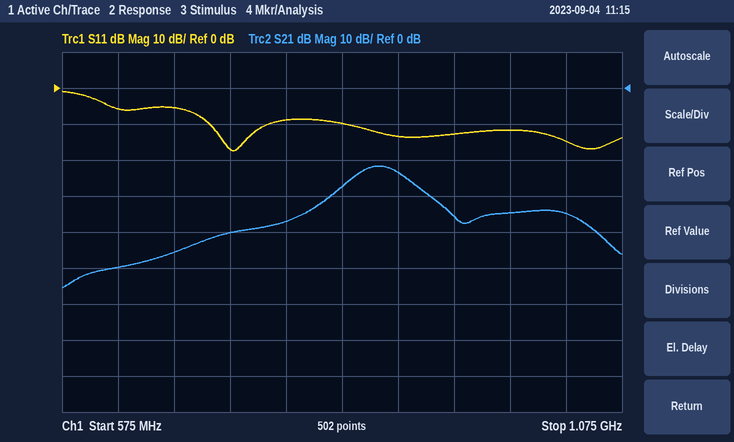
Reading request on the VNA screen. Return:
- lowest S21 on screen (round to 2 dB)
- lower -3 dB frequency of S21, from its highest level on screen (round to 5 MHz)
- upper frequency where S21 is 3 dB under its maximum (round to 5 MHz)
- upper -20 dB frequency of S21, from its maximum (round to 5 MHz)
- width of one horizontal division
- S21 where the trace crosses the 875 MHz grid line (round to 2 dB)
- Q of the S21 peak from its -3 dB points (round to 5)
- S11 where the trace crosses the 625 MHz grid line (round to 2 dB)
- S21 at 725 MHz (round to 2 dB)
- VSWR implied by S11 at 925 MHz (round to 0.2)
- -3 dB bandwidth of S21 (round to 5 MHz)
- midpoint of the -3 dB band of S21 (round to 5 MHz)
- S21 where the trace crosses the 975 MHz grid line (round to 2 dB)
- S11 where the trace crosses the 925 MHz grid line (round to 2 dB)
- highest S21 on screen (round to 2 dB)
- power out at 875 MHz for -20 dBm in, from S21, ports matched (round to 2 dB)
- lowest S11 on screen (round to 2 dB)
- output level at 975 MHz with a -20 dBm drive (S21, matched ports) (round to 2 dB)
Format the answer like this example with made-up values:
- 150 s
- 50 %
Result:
- -56 dB
- 835 MHz
- 880 MHz
- 1.060 GHz
- 50 MHz
- -24 dB
- 20
- -6 dB
- -40 dB
- 1.6
- 45 MHz
- 860 MHz
- -34 dB
- -12 dB
- -22 dB
- -44 dBm
- -18 dB
- -54 dBm
